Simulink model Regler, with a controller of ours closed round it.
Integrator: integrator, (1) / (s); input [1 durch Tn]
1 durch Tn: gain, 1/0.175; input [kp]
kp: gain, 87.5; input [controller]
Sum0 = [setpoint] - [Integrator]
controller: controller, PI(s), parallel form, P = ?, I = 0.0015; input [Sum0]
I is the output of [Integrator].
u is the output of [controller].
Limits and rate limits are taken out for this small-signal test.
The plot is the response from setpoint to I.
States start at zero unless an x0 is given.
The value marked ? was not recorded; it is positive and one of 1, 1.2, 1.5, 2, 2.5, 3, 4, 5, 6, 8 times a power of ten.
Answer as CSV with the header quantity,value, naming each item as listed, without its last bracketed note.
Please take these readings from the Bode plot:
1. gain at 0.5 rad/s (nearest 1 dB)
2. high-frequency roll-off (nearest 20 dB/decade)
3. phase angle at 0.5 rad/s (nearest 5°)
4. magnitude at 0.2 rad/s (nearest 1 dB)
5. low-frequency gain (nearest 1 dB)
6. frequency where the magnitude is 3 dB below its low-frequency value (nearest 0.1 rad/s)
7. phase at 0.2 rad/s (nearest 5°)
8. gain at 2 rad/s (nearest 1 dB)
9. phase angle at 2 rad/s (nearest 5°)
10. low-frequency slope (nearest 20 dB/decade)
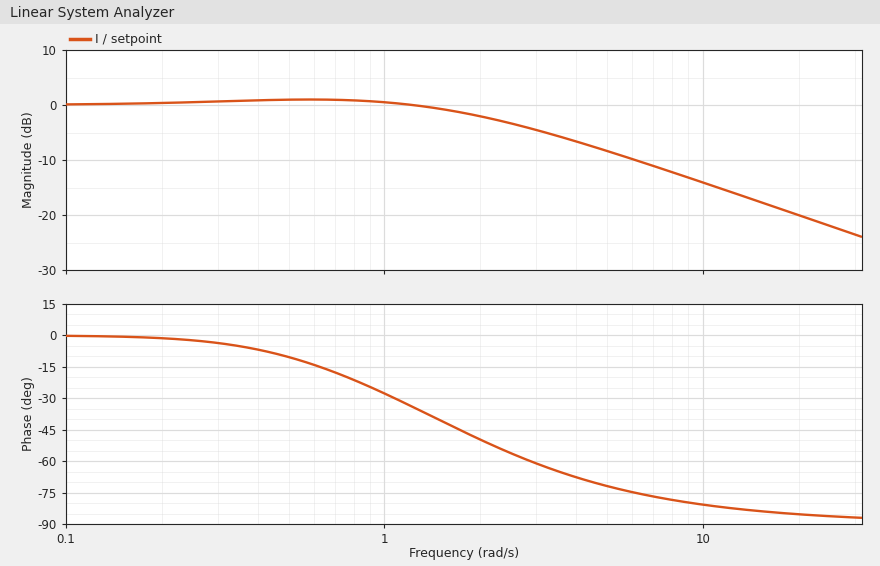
quantity,value
gain at 0.5 rad/s,1 dB
high-frequency roll-off,-20 dB/decade
phase angle at 0.5 rad/s,-10°
magnitude at 0.2 rad/s,0 dB
low-frequency gain,0 dB
frequency where the magnitude is 3 dB below its low-frequency value,2.3 rad/s
phase at 0.2 rad/s,0°
gain at 2 rad/s,-2 dB
phase angle at 2 rad/s,-50°
low-frequency slope,0 dB/decade
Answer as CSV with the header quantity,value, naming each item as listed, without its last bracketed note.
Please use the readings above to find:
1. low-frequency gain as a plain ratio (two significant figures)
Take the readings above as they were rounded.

quantity,value
low-frequency gain as a plain ratio,1.0
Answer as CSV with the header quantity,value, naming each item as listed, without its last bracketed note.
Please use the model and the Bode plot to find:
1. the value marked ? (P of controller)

quantity,value
the value marked ?,0.004
